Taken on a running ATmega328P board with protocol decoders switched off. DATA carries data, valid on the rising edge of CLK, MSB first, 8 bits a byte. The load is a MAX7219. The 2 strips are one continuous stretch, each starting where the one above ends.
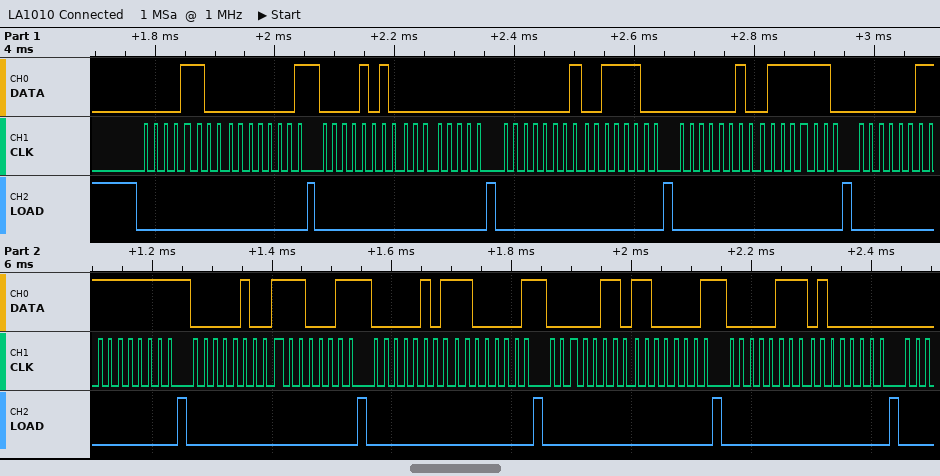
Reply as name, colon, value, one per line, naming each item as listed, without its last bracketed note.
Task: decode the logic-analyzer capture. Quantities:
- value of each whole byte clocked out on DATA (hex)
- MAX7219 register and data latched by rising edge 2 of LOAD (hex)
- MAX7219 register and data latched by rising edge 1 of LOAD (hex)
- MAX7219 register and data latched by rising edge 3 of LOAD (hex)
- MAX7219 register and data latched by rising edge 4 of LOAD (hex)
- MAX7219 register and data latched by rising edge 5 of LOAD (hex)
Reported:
value of each whole byte clocked out on DATA: 0C 01 0A 00 01 3C 02 7E 03 FF 04 E3 05 C1 06 C1 07 40
MAX7219 register and data latched by rising edge 2 of LOAD: register 0xA, data 0x00
MAX7219 register and data latched by rising edge 1 of LOAD: register 0xC, data 0x01
MAX7219 register and data latched by rising edge 3 of LOAD: register 0x1, data 0x3C
MAX7219 register and data latched by rising edge 4 of LOAD: register 0x2, data 0x7E
MAX7219 register and data latched by rising edge 5 of LOAD: register 0x3, data 0xFF
